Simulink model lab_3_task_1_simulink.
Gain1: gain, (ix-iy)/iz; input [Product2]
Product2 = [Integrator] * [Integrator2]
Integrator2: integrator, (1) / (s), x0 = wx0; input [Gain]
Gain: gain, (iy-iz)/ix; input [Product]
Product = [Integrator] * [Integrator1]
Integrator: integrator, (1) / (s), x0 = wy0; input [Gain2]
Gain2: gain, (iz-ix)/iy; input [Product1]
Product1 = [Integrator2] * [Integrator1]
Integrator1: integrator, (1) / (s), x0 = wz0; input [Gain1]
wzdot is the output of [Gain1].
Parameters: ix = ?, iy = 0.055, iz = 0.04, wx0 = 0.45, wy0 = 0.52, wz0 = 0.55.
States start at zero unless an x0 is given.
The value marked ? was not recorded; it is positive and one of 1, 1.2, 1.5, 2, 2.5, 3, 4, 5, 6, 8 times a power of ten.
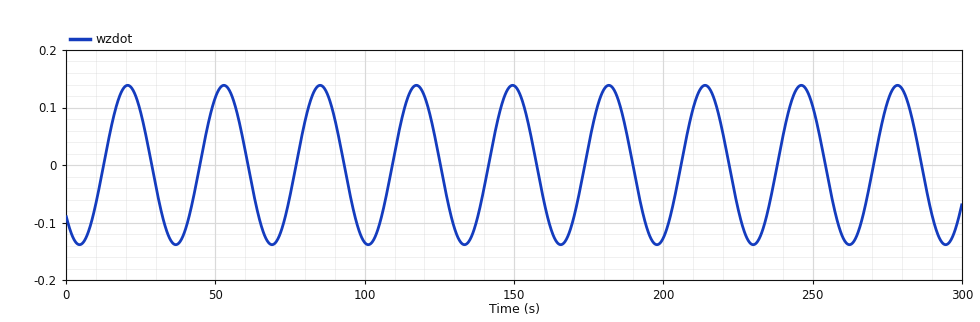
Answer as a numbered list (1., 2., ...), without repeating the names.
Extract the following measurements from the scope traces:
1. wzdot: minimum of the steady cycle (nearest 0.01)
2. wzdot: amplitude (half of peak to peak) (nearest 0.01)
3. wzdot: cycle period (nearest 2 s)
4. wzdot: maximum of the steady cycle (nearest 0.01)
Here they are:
1. -0.14
2. 0.14
3. 32 s
4. 0.14
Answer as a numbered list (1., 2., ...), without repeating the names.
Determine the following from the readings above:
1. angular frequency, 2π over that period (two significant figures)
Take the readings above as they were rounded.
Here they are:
1. 0.20 rad/s
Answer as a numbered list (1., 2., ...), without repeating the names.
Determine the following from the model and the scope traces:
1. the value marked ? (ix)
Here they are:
1. 0.04
